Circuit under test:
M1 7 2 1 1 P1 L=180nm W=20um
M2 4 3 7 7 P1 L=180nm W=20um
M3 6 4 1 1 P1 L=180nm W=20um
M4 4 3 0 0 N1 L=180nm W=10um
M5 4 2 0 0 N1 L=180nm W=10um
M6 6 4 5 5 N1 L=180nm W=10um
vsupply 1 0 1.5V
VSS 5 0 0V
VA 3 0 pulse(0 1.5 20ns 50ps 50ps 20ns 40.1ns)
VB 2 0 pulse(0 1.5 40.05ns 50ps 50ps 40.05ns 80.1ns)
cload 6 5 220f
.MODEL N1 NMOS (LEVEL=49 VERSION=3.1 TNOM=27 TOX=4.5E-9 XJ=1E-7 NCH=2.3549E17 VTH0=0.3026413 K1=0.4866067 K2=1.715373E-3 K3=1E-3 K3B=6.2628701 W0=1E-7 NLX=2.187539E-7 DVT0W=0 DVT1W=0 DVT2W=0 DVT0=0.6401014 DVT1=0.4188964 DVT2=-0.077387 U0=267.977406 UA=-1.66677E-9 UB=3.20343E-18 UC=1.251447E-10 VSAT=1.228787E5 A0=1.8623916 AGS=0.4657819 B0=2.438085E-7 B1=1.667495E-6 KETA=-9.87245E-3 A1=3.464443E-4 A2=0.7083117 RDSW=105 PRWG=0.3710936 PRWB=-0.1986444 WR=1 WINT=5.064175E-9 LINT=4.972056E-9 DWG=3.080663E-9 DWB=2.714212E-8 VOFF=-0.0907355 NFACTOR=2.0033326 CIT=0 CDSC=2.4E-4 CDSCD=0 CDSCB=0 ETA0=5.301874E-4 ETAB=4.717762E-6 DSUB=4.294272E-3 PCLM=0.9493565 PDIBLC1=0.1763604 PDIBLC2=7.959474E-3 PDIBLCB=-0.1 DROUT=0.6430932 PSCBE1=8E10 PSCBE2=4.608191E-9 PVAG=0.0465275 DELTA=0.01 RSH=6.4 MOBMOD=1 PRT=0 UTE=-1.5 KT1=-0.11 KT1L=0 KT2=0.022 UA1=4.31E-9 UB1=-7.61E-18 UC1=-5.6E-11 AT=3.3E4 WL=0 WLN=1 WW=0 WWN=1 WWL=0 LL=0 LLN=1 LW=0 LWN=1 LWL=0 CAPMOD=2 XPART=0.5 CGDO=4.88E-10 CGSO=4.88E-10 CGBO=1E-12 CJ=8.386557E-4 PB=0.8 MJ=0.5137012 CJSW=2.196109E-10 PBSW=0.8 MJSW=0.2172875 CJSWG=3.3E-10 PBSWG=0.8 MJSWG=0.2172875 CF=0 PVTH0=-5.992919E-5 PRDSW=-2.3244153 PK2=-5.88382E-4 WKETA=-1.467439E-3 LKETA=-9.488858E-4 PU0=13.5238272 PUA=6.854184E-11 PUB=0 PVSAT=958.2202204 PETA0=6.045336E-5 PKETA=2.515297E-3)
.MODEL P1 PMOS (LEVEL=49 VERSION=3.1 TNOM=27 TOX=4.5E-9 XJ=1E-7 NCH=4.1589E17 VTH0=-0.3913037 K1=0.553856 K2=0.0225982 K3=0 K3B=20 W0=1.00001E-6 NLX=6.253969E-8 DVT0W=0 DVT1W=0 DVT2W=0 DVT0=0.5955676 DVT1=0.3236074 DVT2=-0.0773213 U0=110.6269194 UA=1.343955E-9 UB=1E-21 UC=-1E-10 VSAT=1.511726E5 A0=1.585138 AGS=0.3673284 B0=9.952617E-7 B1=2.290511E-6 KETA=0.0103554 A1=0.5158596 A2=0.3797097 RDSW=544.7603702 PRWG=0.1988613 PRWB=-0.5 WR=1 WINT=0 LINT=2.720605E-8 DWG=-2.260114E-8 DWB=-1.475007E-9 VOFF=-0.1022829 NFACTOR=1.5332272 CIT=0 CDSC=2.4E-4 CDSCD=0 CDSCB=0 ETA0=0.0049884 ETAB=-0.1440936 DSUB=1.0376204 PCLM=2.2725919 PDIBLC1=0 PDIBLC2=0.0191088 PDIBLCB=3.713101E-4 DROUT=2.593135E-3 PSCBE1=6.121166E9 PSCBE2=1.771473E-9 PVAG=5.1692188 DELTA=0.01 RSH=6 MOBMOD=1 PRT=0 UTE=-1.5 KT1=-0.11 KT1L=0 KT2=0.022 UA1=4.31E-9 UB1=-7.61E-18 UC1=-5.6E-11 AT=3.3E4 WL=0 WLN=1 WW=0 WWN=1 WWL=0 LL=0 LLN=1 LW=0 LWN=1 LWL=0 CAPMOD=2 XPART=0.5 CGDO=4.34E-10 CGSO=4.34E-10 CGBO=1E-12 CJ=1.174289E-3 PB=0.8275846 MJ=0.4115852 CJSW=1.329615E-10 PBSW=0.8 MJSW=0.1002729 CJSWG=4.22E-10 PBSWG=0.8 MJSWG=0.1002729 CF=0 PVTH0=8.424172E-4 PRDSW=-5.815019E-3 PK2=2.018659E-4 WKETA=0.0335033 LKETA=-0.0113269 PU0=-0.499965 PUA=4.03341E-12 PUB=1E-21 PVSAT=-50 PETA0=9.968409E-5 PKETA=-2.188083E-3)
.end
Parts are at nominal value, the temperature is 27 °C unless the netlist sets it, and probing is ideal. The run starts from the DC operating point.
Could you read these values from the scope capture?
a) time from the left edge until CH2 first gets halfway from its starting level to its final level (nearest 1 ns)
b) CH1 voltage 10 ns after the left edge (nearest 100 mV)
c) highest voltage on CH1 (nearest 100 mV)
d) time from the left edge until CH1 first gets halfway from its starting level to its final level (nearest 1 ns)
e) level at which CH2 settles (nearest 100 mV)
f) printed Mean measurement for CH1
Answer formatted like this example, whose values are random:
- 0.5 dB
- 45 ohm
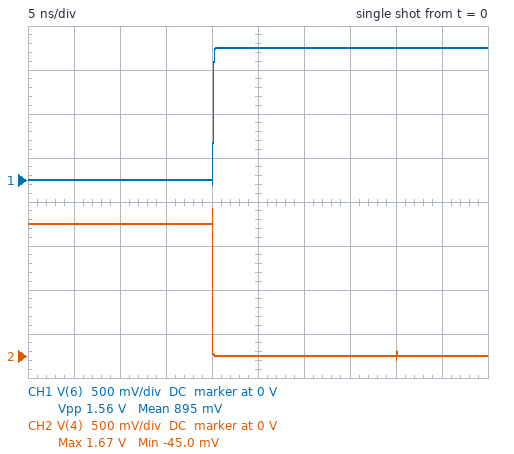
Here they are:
- 20 ns
- 0 V
- 1.5 V
- 20 ns
- 0 V
- 895 mV
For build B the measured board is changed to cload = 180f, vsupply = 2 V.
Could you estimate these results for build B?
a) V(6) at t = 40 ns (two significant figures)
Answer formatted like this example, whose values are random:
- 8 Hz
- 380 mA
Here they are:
- 2.0 V
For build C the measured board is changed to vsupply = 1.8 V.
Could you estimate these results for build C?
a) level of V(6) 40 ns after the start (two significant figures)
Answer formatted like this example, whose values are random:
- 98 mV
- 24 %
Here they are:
- 1.8 V
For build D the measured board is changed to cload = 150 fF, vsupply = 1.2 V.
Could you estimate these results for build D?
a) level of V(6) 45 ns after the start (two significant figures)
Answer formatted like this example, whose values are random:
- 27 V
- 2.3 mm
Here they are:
- 1.2 V
